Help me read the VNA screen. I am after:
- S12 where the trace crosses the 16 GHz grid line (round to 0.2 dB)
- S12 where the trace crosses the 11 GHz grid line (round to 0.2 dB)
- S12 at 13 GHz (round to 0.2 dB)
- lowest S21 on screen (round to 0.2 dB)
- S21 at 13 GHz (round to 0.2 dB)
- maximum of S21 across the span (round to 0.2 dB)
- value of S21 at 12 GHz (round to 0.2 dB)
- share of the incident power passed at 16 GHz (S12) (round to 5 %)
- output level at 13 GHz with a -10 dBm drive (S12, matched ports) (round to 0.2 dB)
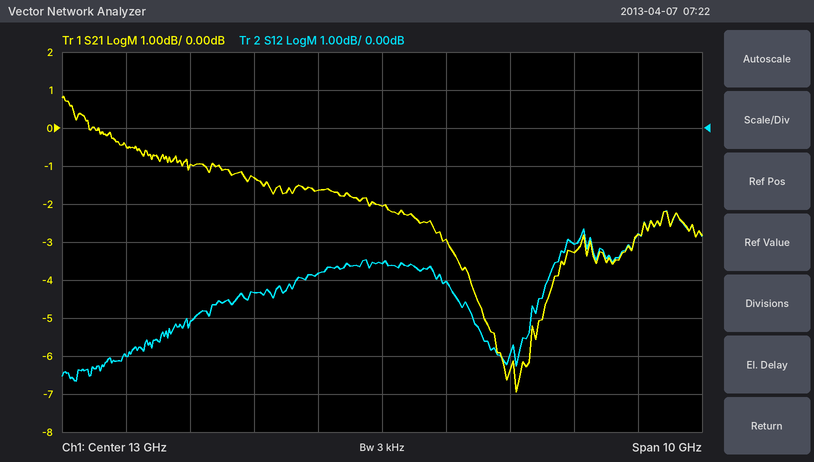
-3.0 dB
-4.4 dB
-3.6 dB
-7.0 dB
-2.0 dB
0.8 dB
-1.6 dB
50 %
-13.6 dBm
